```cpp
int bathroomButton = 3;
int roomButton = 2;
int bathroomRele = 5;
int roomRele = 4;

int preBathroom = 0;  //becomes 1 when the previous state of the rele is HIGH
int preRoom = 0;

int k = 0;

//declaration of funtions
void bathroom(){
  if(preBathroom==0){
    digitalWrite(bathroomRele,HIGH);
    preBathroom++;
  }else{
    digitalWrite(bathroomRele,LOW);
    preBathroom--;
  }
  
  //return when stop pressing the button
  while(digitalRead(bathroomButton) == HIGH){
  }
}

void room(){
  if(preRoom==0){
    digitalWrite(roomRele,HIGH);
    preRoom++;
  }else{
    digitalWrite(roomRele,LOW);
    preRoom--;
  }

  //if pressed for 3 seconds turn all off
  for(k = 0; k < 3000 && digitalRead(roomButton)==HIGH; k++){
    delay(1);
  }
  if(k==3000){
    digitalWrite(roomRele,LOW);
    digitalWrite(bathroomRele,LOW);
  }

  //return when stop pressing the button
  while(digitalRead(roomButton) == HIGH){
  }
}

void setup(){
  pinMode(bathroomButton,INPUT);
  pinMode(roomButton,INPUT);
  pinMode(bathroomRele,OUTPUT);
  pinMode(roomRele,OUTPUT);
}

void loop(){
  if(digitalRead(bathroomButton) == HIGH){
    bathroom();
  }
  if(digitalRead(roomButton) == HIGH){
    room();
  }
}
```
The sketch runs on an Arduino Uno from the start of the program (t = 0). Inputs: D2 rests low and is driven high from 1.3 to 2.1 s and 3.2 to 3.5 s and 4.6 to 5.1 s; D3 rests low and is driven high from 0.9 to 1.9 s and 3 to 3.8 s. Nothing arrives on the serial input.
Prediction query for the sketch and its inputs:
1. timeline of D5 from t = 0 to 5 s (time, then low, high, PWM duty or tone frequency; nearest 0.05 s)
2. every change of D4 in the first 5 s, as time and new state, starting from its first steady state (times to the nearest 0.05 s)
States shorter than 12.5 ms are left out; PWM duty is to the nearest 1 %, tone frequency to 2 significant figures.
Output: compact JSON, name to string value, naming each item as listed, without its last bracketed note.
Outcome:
{"timeline of D5 from t = 0 to 5 s": "0 s low; 0.9 s high; 3 s low", "every change of D4 in the first 5 s, as time and new state, starting from its first steady state": "0 s low; 1.9 s high; 4.6 s low"}
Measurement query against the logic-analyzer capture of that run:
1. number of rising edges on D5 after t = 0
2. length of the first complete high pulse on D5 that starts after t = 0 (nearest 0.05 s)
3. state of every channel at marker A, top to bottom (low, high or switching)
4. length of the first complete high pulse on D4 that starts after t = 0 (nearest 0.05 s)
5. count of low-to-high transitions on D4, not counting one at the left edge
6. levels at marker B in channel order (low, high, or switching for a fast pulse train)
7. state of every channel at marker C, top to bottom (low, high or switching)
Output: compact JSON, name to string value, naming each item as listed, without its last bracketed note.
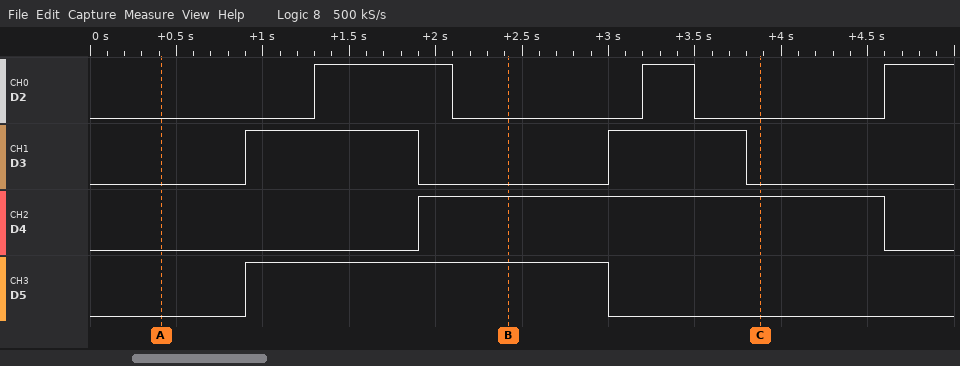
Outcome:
{"number of rising edges on D5 after t = 0": "1", "length of the first complete high pulse on D5 that starts after t = 0": "2.10 s", "state of every channel at marker A, top to bottom": "D2 low, D3 low, D4 low, D5 low", "length of the first complete high pulse on D4 that starts after t = 0": "2.70 s", "count of low-to-high transitions on D4, not counting one at the left edge": "1", "levels at marker B in channel order": "D2 low, D3 low, D4 high, D5 high", "state of every channel at marker C, top to bottom": "D2 low, D3 low, D4 high, D5 low"}
